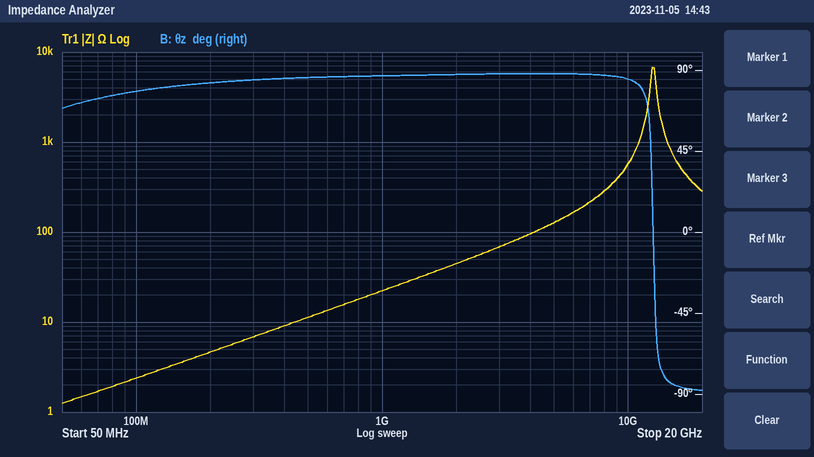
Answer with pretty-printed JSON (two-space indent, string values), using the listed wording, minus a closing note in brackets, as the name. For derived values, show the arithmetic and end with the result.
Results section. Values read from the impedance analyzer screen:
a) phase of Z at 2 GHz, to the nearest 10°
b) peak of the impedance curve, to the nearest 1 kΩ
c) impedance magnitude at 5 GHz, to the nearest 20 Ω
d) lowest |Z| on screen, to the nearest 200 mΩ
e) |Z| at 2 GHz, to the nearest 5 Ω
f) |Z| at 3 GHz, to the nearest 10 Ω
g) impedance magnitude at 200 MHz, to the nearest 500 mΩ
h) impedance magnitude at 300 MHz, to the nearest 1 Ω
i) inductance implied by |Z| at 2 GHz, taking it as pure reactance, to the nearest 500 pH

{
  "phase of Z at 2 GHz, to the nearest 10°": "90°",
  "peak of the impedance curve, to the nearest 1 kΩ": "7 kΩ",
  "impedance magnitude at 5 GHz, to the nearest 20 Ω": "120 Ω",
  "lowest |Z| on screen, to the nearest 200 mΩ": "1.2 Ω",
  "|Z| at 2 GHz, to the nearest 5 Ω": "45 Ω",
  "|Z| at 3 GHz, to the nearest 10 Ω": "70 Ω",
  "impedance magnitude at 200 MHz, to the nearest 500 mΩ": "4.5 Ω",
  "impedance magnitude at 300 MHz, to the nearest 1 Ω": "7 Ω",
  "inductance implied by |Z| at 2 GHz, taking it as pure reactance, to the nearest 500 pH": "L = 45 Ω/(2π × 2 GHz) ≈ 3.58 nH, so 3.5 nH to the nearest 500 pH"
}
